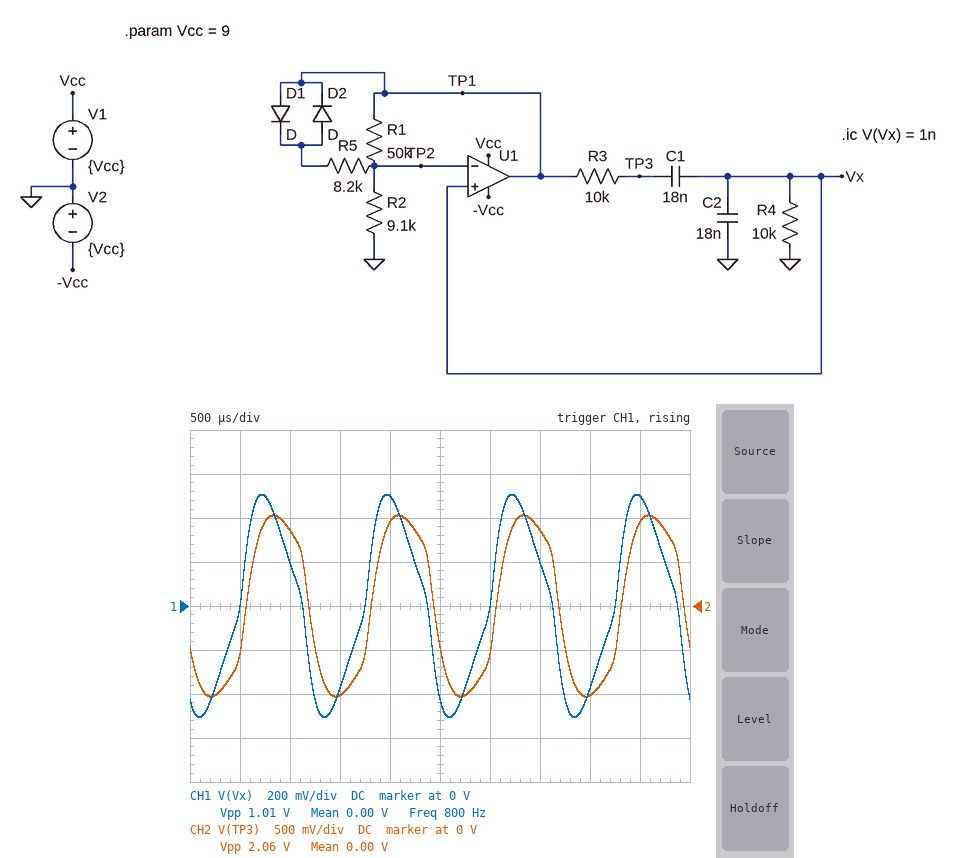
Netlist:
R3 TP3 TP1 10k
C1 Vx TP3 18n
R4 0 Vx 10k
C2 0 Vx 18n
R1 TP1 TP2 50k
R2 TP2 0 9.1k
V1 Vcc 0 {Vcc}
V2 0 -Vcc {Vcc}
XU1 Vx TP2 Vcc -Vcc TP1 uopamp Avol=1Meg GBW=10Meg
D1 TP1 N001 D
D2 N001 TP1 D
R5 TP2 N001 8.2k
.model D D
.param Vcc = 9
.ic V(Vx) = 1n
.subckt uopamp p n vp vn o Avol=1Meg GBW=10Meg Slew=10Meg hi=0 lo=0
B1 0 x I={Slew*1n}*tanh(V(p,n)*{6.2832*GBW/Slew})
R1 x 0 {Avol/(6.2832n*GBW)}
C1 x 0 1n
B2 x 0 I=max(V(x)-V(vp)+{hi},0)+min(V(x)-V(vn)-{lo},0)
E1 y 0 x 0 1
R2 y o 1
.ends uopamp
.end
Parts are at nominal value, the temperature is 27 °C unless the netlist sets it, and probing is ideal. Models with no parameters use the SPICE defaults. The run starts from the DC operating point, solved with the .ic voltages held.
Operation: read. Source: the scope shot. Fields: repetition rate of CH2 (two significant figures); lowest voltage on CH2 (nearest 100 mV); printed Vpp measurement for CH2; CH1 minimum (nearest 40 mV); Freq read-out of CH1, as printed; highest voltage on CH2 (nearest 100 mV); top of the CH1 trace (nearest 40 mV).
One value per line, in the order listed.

800 Hz
-1.0 V
2.06 V
-520 mV
800 Hz
1.0 V
520 mV
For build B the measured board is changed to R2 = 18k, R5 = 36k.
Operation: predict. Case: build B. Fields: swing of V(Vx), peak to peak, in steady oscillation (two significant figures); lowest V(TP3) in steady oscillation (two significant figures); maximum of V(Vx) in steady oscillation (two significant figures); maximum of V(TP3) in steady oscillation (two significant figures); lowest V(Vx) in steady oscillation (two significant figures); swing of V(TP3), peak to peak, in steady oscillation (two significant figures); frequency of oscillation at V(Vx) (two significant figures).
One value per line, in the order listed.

890 mV
-950 mV
450 mV
950 mV
-450 mV
1.9 V
860 Hz
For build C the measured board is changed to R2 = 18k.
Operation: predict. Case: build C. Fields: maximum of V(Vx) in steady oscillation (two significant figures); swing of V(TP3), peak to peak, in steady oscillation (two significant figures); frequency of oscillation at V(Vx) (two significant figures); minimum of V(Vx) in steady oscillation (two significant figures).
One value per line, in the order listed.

330 mV
1.4 V
840 Hz
-330 mV
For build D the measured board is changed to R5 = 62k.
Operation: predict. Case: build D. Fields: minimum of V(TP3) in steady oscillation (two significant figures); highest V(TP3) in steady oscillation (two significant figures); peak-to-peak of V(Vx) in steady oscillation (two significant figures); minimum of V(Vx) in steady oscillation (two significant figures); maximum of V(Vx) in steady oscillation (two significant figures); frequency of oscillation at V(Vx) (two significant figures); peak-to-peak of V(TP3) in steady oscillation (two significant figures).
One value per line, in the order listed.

-7.7 V
7.7 V
7.4 V
-3.7 V
3.7 V
750 Hz
15 V
